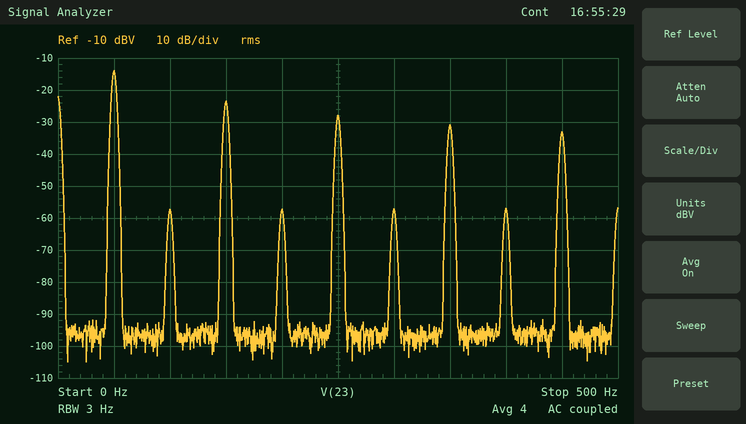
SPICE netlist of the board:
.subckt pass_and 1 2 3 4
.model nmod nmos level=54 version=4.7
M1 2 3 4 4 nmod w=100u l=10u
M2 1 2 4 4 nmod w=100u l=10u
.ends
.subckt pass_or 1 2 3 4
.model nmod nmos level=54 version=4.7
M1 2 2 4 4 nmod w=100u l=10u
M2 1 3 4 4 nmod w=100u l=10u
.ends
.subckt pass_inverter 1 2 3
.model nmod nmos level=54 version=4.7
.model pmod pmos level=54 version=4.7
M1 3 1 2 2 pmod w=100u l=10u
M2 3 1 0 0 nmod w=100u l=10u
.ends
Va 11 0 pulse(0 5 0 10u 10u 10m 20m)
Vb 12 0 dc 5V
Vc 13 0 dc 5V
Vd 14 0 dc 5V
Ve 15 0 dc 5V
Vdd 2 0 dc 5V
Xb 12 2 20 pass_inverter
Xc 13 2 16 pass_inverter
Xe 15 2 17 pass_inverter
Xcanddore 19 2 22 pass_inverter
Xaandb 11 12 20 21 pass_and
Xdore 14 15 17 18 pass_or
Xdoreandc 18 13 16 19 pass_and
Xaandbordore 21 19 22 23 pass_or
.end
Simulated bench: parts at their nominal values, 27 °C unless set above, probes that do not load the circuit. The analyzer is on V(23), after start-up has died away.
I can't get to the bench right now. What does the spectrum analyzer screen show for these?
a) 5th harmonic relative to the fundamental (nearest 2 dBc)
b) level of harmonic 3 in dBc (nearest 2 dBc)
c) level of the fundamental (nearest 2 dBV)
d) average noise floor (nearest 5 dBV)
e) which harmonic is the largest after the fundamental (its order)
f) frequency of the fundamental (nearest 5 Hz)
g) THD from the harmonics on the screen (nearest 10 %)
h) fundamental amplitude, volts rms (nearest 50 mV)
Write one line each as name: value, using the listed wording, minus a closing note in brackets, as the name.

5th harmonic relative to the fundamental: -14 dBc
level of harmonic 3 in dBc: -10 dBc
level of the fundamental: -14 dBV
average noise floor: -95 dBV
which harmonic is the largest after the fundamental: 3
frequency of the fundamental: 50 Hz
THD from the harmonics on the screen: 40 %
fundamental amplitude, volts rms: 200 mV
